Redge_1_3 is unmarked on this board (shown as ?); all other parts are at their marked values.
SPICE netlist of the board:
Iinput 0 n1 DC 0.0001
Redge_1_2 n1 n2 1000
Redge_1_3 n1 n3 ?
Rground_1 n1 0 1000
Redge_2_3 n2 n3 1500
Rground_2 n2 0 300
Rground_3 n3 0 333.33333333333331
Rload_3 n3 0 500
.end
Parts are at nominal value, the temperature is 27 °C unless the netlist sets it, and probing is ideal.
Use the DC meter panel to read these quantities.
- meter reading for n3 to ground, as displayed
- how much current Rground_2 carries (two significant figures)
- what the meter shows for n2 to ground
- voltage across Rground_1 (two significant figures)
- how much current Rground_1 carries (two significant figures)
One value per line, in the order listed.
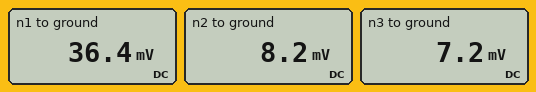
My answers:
7.2 mV
27 µA
8.2 mV
36 mV
36 µA
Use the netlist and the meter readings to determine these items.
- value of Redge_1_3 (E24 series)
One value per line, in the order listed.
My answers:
820 Ω
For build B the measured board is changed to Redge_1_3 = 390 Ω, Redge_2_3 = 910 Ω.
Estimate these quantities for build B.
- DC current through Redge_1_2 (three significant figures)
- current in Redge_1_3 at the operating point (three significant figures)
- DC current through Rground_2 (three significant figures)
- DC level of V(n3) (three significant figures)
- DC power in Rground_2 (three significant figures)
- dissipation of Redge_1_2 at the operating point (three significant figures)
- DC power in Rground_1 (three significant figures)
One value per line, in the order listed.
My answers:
21.6 µA
49.6 µA
24.0 µA
9.44 mV
173 nW
466 nW
829 nW
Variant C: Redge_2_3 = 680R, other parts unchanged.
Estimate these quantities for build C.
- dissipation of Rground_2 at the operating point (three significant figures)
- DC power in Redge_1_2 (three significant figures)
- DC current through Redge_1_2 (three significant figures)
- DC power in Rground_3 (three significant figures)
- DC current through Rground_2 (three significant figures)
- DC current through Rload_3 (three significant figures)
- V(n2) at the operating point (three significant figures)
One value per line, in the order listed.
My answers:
220 nW
797 nW
28.2 µA
161 nW
27.1 µA
14.6 µA
8.12 mV
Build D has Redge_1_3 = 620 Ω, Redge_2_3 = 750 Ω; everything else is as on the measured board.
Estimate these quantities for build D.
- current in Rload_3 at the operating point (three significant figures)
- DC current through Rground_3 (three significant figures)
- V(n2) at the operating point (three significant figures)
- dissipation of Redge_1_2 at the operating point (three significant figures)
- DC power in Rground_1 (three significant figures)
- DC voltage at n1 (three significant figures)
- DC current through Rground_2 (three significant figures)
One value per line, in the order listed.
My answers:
16.2 µA
24.3 µA
7.81 mV
658 nW
1.12 µW
33.5 mV
26.0 µA
